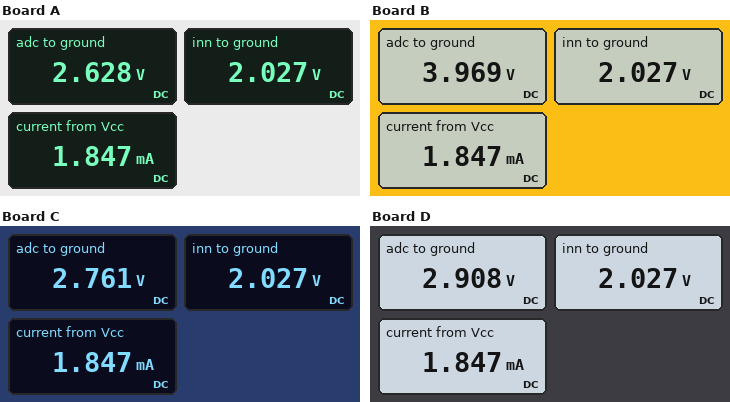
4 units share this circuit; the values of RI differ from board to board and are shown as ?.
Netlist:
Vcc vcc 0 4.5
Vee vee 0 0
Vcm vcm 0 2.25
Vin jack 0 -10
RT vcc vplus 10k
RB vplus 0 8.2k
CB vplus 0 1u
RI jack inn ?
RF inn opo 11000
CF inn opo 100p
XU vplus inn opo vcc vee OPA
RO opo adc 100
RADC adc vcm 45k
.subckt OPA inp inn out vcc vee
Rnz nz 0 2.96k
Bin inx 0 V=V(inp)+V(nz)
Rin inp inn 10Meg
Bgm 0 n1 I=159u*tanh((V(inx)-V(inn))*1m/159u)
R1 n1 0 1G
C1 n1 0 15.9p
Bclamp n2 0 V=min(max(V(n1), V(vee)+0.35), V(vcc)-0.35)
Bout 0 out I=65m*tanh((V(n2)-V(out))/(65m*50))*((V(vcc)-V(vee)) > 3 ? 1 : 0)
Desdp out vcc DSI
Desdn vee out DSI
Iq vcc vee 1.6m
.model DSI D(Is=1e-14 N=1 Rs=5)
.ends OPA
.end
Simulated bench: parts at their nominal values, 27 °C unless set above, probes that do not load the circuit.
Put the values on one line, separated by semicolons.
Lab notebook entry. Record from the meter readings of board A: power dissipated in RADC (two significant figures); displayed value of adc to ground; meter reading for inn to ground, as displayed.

3.2 µW; 2.628 V; 2.027 V
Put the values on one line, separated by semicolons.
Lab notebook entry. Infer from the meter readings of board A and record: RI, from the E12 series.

220 kΩ
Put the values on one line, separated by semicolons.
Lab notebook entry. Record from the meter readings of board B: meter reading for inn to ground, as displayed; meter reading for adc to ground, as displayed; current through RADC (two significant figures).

2.027 V; 3.969 V; 38 µA
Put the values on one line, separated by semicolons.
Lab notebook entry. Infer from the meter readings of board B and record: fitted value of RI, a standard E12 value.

68 kΩ
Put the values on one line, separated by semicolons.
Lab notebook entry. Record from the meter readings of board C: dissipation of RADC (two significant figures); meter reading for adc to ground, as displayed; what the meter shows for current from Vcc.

5.8 µW; 2.761 V; 1.847 mA
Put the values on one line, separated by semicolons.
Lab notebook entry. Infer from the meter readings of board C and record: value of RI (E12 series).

180 kΩ
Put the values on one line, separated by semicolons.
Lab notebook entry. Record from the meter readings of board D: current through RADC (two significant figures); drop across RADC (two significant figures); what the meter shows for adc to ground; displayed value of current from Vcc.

15 µA; 660 mV; 2.908 V; 1.847 mA
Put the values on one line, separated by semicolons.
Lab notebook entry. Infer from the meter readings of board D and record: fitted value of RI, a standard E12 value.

150 kΩ
